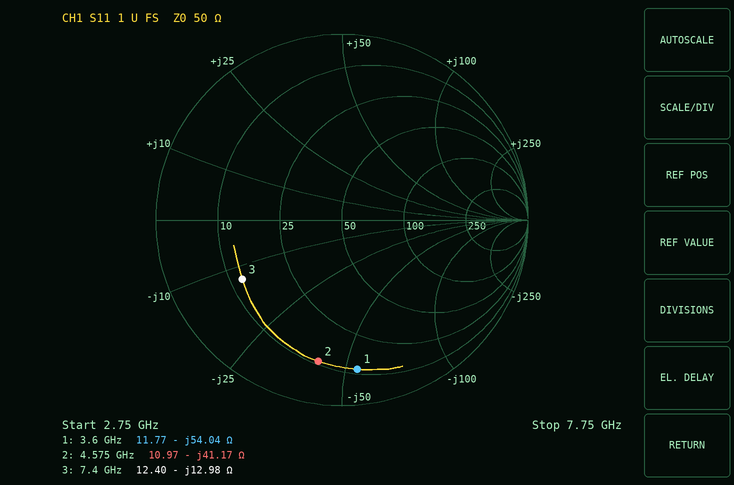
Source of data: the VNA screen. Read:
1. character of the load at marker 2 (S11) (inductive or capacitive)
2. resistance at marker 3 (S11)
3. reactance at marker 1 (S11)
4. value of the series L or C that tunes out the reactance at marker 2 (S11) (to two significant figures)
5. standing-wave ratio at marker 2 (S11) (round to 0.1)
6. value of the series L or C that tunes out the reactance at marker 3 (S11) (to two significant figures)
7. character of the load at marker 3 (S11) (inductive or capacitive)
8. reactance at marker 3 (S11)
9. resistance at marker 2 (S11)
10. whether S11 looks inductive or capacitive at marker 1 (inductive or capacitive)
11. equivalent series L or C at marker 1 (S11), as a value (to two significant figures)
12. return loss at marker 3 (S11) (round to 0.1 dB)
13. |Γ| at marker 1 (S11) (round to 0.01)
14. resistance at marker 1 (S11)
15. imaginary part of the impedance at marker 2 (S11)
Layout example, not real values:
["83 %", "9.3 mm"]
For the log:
["capacitive", "12.40 Ω", "-54.04 Ω", "1.4 nH", "7.7", "280 pH", "capacitive", "-12.98 Ω", "10.97 Ω", "capacitive", "820 fF", "4.1 dB", "0.81", "11.77 Ω", "-41.17 Ω"]
